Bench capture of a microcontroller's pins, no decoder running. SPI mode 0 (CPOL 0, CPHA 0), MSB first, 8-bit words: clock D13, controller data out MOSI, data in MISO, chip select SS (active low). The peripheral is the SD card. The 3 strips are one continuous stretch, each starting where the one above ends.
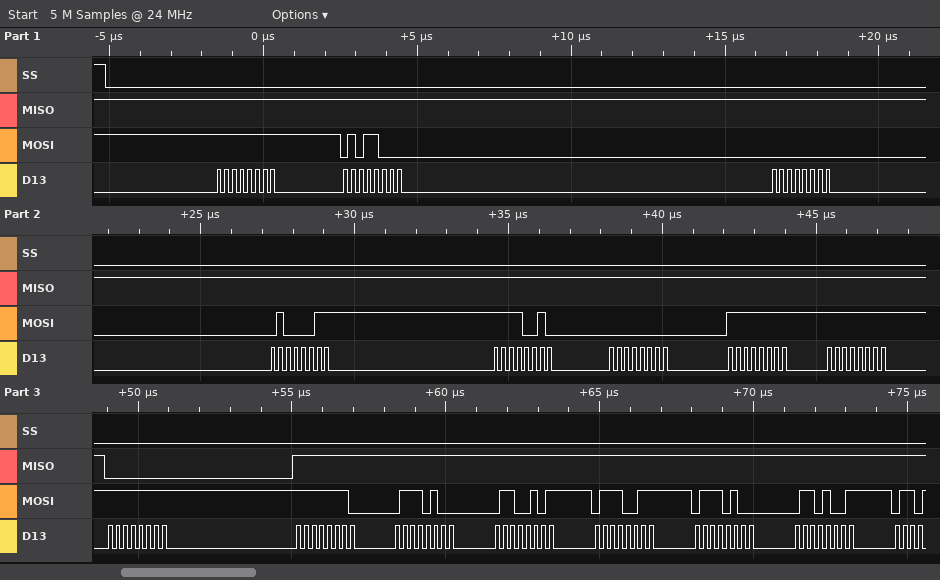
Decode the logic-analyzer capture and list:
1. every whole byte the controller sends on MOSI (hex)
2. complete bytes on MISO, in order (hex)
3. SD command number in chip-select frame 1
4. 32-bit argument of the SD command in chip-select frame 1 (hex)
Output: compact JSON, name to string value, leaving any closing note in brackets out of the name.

{"every whole byte the controller sends on MOSI": "0xFF 0x58 0x00 0x43 0xF2 0x00 0xFF 0xFF 0xFF 0xFE 0x74 0x65 0x73 0x74 0x69", "complete bytes on MISO, in order": "0xFF 0xFF 0xFF 0xFF 0xFF 0xFF 0xFF 0xFF 0x00 0xFF 0xFF 0xFF 0xFF 0xFF 0xFF", "SD command number in chip-select frame 1": "CMD24", "32-bit argument of the SD command in chip-select frame 1": "0x0043F200"}
